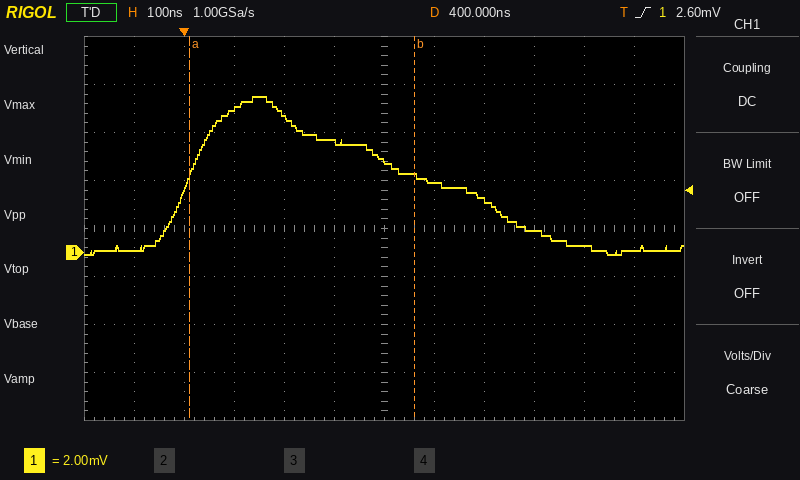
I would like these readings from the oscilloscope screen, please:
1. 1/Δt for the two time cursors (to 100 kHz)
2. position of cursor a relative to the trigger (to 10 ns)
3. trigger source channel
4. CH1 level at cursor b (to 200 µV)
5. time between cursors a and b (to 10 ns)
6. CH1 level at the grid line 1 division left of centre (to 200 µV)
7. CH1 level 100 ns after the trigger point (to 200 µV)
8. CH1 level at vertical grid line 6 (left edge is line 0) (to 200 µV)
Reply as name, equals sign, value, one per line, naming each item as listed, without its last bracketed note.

1/Δt for the two time cursors = 2.2 MHz
position of cursor a relative to the trigger = +10 ns
trigger source channel = CH1
CH1 level at cursor b = 3.2 mV
time between cursors a and b = 450 ns
CH1 level at the grid line 1 division left of centre = 4.6 mV
CH1 level 100 ns after the trigger point = 6.0 mV
CH1 level at vertical grid line 6 (left edge is line 0) = 3.8 mV
